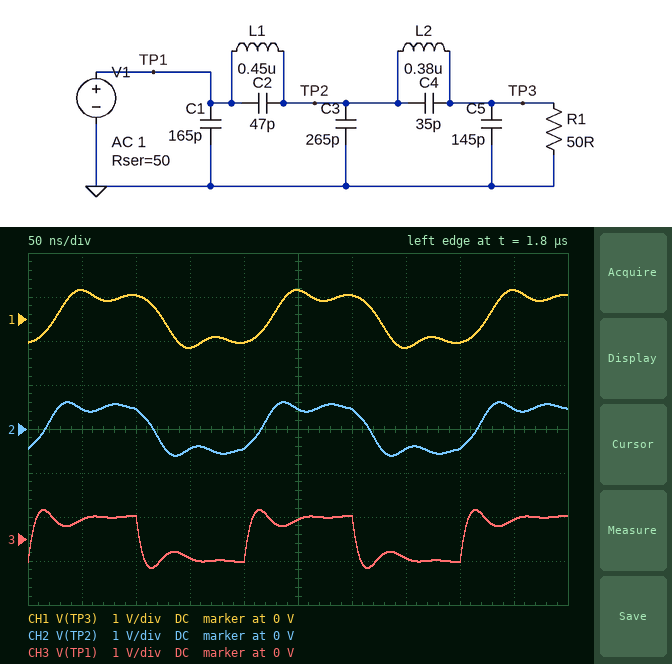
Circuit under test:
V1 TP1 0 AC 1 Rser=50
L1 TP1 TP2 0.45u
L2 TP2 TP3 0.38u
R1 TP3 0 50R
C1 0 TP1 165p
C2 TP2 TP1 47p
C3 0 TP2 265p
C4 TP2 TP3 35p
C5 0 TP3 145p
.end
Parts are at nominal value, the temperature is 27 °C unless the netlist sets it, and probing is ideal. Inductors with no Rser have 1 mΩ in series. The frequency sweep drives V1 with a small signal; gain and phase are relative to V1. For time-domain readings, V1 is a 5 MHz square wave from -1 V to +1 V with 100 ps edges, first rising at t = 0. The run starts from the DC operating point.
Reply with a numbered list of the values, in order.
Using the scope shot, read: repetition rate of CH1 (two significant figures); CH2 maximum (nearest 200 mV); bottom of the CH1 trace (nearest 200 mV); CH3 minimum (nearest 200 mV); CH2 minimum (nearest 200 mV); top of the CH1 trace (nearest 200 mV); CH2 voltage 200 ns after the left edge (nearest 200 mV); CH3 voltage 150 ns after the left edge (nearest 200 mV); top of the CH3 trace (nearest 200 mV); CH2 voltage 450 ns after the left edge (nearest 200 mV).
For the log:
1. 5.0 MHz
2. 600 mV
3. -600 mV
4. -600 mV
5. -600 mV
6. 600 mV
7. -400 mV
8. -400 mV
9. 600 mV
10. 400 mV
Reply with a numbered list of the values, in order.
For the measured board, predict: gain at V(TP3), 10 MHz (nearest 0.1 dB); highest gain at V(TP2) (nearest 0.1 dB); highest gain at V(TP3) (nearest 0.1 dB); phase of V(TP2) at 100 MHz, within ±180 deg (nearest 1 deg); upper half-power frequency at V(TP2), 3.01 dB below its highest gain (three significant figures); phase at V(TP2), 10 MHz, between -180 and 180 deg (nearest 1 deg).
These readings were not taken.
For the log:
1. -6.1 dB
2. -4.9 dB
3. -6.0 dB
4. -81 deg
5. 23.3 MHz
6. -50 deg
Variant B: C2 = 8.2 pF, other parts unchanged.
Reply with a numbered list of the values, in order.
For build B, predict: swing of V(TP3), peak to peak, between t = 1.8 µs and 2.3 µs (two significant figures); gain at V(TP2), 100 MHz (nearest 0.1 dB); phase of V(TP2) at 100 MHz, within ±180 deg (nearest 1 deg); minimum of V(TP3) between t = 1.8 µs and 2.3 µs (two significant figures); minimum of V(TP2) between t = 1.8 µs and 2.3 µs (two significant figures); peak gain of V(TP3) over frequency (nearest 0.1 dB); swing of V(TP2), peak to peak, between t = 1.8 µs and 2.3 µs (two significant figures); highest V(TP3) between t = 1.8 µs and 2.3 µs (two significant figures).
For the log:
1. 1.4 V
2. -55.7 dB
3. -79 deg
4. -680 mV
5. -670 mV
6. -6.0 dB
7. 1.3 V
8. 680 mV
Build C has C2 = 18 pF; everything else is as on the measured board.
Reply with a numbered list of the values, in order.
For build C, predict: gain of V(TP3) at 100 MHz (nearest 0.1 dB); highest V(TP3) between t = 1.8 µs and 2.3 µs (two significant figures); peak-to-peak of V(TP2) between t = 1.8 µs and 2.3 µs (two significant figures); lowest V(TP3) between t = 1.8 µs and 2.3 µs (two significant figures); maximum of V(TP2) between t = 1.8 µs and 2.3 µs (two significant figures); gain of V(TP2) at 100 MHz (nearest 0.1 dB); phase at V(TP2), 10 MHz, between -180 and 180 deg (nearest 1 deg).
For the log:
1. -58.6 dB
2. 680 mV
3. 1.3 V
4. -680 mV
5. 650 mV
6. -42.8 dB
7. -49 deg
